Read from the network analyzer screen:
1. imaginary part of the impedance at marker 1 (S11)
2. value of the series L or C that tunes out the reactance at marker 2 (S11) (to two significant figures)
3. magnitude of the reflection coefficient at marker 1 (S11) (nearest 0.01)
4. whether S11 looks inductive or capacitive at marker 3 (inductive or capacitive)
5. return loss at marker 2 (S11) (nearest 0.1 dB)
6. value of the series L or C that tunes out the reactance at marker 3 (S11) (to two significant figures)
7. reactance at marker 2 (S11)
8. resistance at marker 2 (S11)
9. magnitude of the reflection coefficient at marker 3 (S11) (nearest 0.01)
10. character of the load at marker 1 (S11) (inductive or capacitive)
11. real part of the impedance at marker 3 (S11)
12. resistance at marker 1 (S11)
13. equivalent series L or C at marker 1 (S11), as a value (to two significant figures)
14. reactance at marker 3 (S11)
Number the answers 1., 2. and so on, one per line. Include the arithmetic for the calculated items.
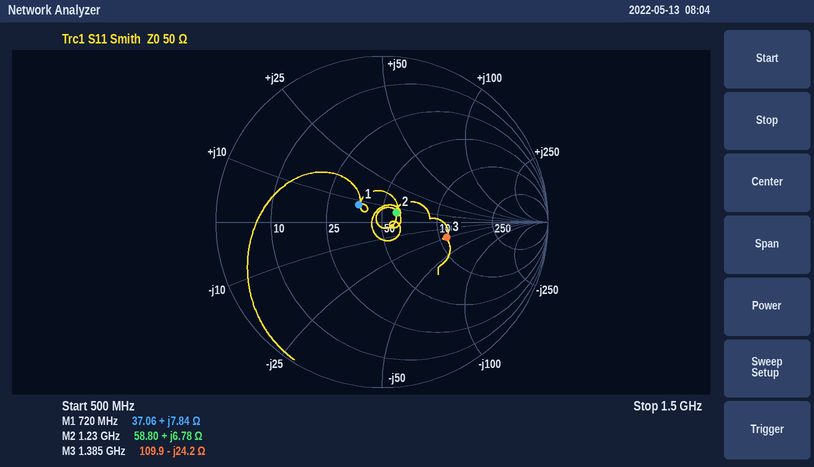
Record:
1. +7.84 Ω
2. C = 1/(2π × 1.23 GHz × 6.78 Ω) ≈ 19 pF
3. 0.17
4. capacitive
5. 19.8 dB
6. L = 24.2 Ω/(2π × 1.385 GHz) ≈ 2.8 nH
7. +6.78 Ω
8. 58.80 Ω
9. 0.40
10. inductive
11. 109.9 Ω
12. 37.06 Ω
13. L = 7.84 Ω/(2π × 720 MHz) ≈ 1.7 nH
14. -24.2 Ω
